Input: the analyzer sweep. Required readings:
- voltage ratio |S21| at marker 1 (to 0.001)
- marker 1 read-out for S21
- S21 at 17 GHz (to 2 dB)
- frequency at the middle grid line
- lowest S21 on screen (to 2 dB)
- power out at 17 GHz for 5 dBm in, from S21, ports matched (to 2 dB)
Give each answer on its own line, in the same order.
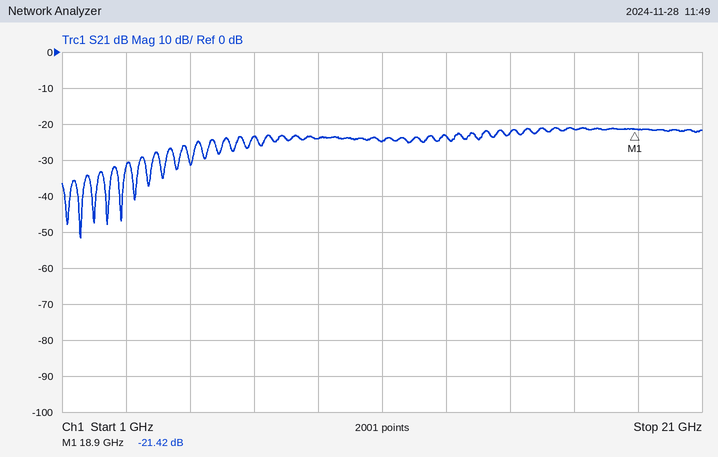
0.085
-21.42 dB
-22 dB
11 GHz
-52 dB
-16 dBm
